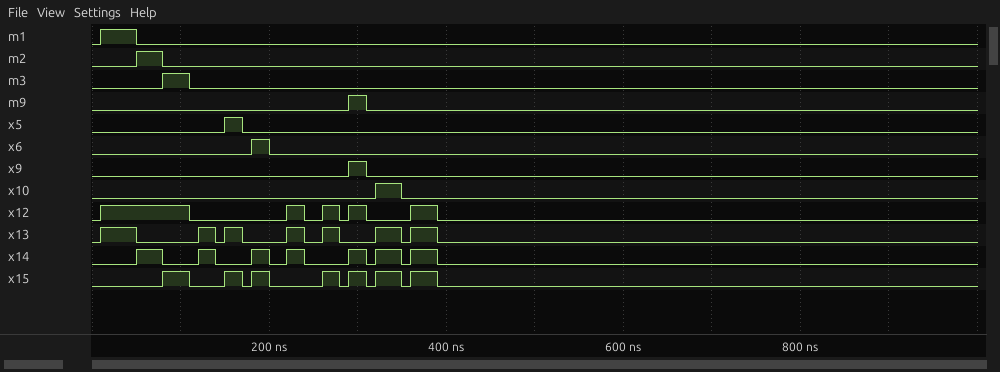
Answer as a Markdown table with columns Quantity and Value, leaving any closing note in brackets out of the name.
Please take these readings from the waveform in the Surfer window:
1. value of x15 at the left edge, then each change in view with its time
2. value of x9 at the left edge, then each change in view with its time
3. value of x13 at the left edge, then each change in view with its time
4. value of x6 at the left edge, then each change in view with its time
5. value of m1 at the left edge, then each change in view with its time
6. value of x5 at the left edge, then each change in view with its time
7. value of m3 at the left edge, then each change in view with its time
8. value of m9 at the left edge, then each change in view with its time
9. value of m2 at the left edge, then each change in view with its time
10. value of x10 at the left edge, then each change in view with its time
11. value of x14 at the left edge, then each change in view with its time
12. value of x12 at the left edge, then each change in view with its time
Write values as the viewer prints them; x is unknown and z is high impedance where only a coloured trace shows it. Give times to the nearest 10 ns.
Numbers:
| Quantity | Value |
|---|---|
| value of x15 at the left edge, then each change in view with its time | 0, 1 at 80 ns, 0 at 110 ns, 1 at 150 ns, 0 at 170 ns, 1 at 180 ns, 0 at 200 ns, 1 at 260 ns, 0 at 280 ns, 1 at 290 ns, 0 at 310 ns, 1 at 320 ns, 0 at 350 ns, 1 at 360 ns, 0 at 390 ns |
| value of x9 at the left edge, then each change in view with its time | 0, 1 at 290 ns, 0 at 310 ns |
| value of x13 at the left edge, then each change in view with its time | 0, 1 at 10 ns, 0 at 50 ns, 1 at 120 ns, 0 at 140 ns, 1 at 150 ns, 0 at 170 ns, 1 at 220 ns, 0 at 240 ns, 1 at 260 ns, 0 at 280 ns, 1 at 320 ns, 0 at 350 ns, 1 at 360 ns, 0 at 390 ns |
| value of x6 at the left edge, then each change in view with its time | 0, 1 at 180 ns, 0 at 200 ns |
| value of m1 at the left edge, then each change in view with its time | 0, 1 at 10 ns, 0 at 50 ns |
| value of x5 at the left edge, then each change in view with its time | 0, 1 at 150 ns, 0 at 170 ns |
| value of m3 at the left edge, then each change in view with its time | 0, 1 at 80 ns, 0 at 110 ns |
| value of m9 at the left edge, then each change in view with its time | 0, 1 at 290 ns, 0 at 310 ns |
| value of m2 at the left edge, then each change in view with its time | 0, 1 at 50 ns, 0 at 80 ns |
| value of x10 at the left edge, then each change in view with its time | 0, 1 at 320 ns, 0 at 350 ns |
| value of x14 at the left edge, then each change in view with its time | 0, 1 at 50 ns, 0 at 80 ns, 1 at 120 ns, 0 at 140 ns, 1 at 180 ns, 0 at 200 ns, 1 at 220 ns, 0 at 240 ns, 1 at 290 ns, 0 at 310 ns, 1 at 320 ns, 0 at 350 ns, 1 at 360 ns, 0 at 390 ns |
| value of x12 at the left edge, then each change in view with its time | 0, 1 at 10 ns, 0 at 110 ns, 1 at 220 ns, 0 at 240 ns, 1 at 260 ns, 0 at 280 ns, 1 at 290 ns, 0 at 310 ns, 1 at 360 ns, 0 at 390 ns |
